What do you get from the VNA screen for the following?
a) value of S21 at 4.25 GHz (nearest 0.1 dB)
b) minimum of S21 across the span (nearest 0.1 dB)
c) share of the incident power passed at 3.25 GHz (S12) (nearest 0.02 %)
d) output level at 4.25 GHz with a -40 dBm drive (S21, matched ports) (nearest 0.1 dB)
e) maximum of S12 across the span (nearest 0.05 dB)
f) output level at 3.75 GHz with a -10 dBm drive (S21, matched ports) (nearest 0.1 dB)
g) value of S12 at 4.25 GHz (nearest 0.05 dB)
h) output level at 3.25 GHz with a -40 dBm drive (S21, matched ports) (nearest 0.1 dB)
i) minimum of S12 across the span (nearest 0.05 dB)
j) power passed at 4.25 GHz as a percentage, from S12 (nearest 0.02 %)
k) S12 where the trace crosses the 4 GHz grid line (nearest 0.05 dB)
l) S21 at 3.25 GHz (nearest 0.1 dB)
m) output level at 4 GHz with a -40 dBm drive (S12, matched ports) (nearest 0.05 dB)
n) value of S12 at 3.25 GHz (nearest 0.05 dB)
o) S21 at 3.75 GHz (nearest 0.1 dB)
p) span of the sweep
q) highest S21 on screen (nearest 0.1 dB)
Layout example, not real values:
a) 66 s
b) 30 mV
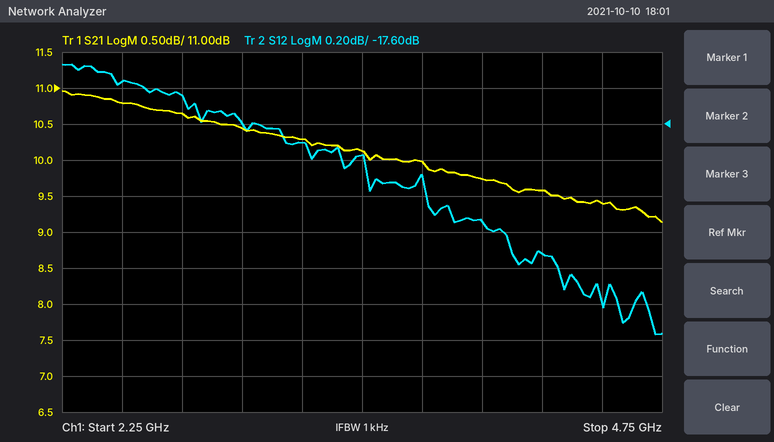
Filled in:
a) 9.6 dB
b) 9.1 dB
c) 1.70 %
d) -30.4 dBm
e) -17.25 dB
f) 0.0 dBm
g) -18.30 dB
h) -29.7 dBm
i) -18.75 dB
j) 1.48 %
k) -18.15 dB
l) 10.3 dB
m) -58.15 dBm
n) -17.70 dB
o) 10.0 dB
p) 2.5 GHz
q) 11.0 dB
